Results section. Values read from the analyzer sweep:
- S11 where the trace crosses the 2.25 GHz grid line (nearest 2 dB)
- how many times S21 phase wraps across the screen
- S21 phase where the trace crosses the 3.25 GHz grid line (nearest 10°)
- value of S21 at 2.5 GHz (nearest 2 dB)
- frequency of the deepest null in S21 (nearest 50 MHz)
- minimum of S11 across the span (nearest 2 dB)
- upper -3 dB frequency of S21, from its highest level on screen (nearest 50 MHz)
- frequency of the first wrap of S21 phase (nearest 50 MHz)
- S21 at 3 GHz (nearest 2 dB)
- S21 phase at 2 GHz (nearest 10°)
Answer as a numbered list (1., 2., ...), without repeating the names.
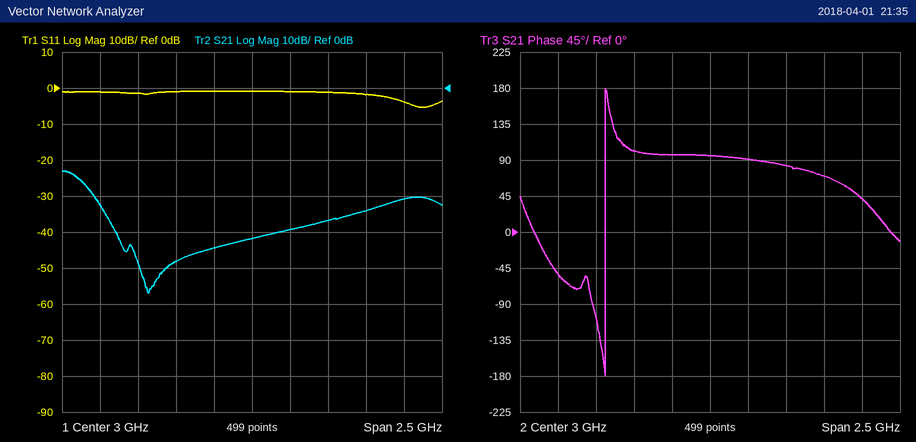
1. -2 dB
2. 1
3. 90°
4. -48 dB
5. 2.30 GHz
6. -6 dB
7. 1.90 GHz
8. 2.30 GHz
9. -42 dB
10. -50°
